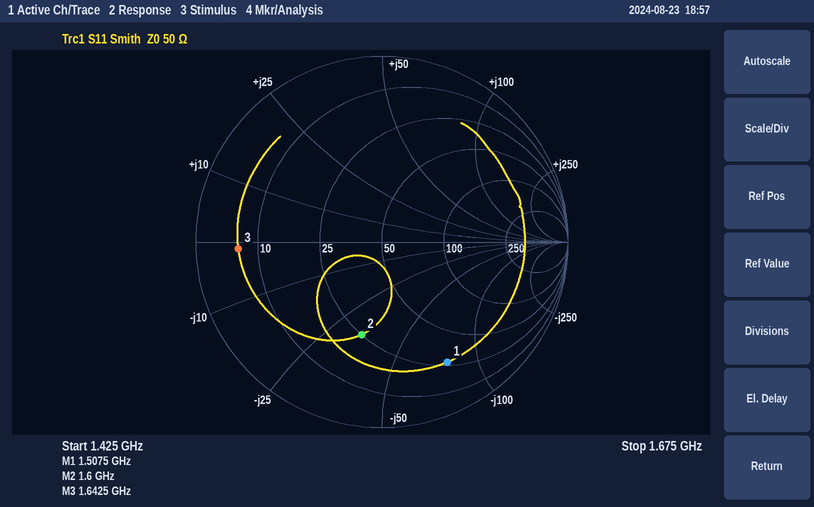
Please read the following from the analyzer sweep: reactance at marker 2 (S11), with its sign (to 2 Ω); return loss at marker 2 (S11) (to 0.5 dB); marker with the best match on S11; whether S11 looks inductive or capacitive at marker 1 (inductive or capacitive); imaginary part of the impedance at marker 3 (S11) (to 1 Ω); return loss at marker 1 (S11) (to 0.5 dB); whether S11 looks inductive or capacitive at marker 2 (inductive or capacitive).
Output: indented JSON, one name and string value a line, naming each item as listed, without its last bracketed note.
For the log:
{
  "reactance at marker 2 (S11), with its sign": "-34 Ω",
  "return loss at marker 2 (S11)": "6.0 dB",
  "marker with the best match on S11": "marker 2",
  "whether S11 looks inductive or capacitive at marker 1": "capacitive",
  "imaginary part of the impedance at marker 3 (S11)": "-1 Ω",
  "return loss at marker 1 (S11)": "2.5 dB",
  "whether S11 looks inductive or capacitive at marker 2": "capacitive"
}
